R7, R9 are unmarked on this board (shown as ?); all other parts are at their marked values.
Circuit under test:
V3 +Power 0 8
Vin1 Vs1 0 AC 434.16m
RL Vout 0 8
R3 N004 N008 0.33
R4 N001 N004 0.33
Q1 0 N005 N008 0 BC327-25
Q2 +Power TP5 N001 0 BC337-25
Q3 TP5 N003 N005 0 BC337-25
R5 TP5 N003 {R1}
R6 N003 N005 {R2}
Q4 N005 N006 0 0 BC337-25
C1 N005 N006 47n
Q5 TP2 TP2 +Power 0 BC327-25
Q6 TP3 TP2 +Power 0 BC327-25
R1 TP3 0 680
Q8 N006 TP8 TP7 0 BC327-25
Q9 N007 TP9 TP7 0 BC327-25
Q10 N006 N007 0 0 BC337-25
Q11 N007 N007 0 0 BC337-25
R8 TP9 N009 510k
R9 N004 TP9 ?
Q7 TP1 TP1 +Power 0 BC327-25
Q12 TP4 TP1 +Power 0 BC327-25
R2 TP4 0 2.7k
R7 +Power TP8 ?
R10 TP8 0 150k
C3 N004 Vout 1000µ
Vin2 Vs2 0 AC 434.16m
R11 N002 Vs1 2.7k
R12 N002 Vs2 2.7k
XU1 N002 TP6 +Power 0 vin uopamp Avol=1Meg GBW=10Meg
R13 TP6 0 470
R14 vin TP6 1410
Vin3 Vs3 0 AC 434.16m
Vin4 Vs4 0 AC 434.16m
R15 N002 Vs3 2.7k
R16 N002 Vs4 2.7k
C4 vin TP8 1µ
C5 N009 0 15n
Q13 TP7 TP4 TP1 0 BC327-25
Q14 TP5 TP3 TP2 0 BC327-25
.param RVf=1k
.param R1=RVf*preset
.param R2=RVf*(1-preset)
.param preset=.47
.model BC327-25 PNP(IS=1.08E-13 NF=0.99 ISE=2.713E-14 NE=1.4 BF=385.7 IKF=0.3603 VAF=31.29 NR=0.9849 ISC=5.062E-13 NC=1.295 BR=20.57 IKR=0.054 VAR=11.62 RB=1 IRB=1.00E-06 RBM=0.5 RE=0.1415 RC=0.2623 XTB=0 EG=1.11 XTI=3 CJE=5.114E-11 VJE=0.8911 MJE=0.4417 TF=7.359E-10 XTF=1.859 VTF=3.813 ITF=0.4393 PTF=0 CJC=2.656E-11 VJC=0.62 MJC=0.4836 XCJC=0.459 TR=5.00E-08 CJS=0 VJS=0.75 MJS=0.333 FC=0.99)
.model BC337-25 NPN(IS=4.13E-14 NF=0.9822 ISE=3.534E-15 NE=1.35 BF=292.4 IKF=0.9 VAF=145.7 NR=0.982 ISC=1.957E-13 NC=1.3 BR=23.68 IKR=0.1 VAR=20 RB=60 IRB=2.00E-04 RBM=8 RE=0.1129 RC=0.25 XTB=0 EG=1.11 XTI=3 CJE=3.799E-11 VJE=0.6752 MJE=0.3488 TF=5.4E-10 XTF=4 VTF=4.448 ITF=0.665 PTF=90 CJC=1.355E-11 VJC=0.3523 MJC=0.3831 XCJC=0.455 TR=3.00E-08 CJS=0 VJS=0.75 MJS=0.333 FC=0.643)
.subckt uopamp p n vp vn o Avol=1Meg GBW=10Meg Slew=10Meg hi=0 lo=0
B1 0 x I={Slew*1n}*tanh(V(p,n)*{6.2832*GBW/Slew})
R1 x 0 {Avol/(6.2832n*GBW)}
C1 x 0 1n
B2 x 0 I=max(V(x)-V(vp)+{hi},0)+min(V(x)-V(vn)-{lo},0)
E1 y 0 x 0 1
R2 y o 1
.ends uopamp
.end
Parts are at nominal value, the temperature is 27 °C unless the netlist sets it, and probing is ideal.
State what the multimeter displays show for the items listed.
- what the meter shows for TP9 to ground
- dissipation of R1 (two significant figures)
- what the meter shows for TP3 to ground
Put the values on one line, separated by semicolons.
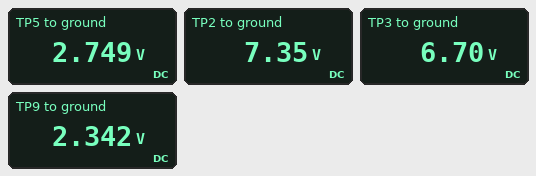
2.342 V; 66 mW; 6.70 V
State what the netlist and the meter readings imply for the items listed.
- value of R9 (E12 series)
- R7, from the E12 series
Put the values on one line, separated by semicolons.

68 kΩ; 470 kΩ
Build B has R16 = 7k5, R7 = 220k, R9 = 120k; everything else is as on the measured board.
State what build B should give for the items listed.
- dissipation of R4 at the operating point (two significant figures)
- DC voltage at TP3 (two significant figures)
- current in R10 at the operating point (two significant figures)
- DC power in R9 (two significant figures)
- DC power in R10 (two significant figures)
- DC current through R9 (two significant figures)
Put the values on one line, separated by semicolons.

5.1 µW; 6.7 V; 24 µA; 1.4 µW; 84 µW; 3.4 µA
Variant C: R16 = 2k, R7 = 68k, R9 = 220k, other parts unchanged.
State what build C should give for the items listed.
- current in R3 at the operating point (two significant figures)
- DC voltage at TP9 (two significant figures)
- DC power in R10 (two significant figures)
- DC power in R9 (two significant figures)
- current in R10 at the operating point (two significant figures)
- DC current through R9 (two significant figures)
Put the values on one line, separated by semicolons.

4.0 mA; 5.7 V; 210 µW; 2.2 µW; 38 µA; 3.2 µA
